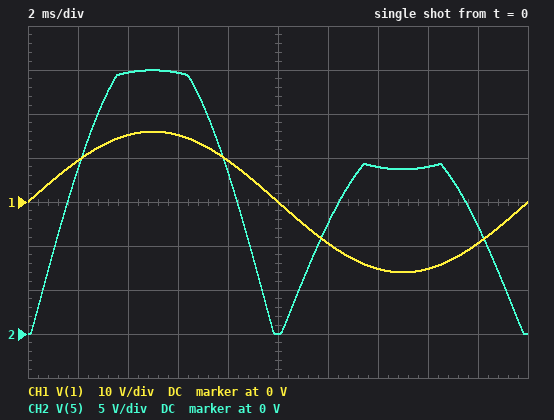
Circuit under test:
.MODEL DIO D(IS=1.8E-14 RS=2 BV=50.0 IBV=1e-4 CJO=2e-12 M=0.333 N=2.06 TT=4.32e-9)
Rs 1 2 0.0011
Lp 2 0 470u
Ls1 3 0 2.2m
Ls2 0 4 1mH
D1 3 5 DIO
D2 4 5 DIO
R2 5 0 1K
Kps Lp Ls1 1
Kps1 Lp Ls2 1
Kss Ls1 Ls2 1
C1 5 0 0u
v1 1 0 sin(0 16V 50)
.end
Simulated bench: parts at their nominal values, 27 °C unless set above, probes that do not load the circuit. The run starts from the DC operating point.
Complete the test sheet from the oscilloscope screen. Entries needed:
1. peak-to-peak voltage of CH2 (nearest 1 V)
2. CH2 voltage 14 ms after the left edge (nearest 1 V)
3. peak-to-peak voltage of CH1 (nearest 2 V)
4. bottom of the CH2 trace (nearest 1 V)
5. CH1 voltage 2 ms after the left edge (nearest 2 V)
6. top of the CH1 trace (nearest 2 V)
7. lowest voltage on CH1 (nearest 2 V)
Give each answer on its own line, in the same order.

30 V
19 V
32 V
0 V
10 V
16 V
-16 V
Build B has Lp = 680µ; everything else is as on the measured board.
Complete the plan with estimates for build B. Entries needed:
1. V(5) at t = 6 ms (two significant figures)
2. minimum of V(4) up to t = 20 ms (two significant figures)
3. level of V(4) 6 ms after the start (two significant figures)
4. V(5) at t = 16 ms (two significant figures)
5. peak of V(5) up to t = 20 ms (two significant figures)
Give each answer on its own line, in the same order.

26 V
-19 V
-18 V
17 V
27 V
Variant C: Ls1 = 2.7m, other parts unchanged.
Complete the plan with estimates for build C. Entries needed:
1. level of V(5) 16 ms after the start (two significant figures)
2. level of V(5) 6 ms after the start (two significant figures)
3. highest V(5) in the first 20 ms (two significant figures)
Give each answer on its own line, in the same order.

17 V
31 V
32 V
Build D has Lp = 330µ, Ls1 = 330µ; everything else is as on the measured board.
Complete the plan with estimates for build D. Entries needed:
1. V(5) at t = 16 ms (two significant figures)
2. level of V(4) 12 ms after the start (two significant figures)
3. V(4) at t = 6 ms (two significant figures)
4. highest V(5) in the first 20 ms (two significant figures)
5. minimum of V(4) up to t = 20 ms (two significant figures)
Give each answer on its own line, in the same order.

25 V
17 V
-26 V
27 V
-28 V
